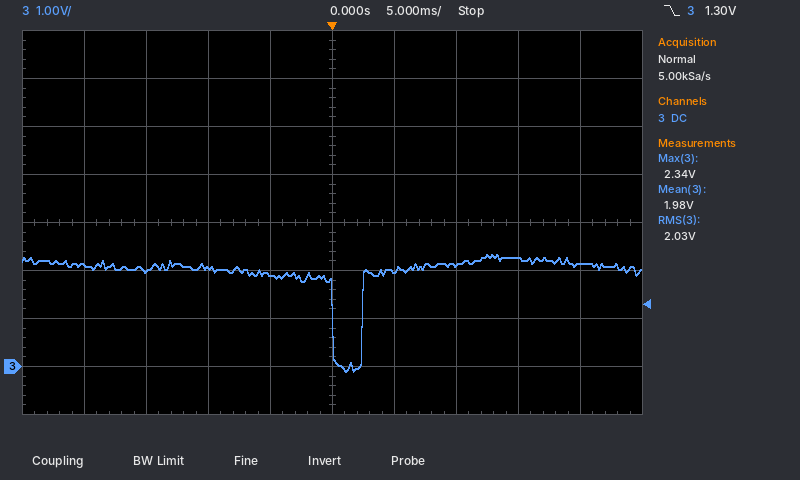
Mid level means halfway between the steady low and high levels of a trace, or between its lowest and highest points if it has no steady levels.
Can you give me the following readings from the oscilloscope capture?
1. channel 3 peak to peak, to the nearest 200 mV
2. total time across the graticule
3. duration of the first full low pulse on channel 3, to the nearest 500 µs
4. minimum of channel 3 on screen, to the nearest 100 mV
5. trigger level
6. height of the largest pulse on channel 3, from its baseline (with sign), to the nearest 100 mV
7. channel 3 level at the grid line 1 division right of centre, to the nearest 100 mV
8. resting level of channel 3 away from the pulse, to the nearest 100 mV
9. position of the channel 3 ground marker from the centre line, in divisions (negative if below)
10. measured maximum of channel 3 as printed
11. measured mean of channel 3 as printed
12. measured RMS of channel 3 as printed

2.4 V
50 ms
2.5 ms
-100 mV
1.30 V
-2.2 V
2.0 V
2.1 V
-3.0 div
2.34 V
1.98 V
2.03 V
